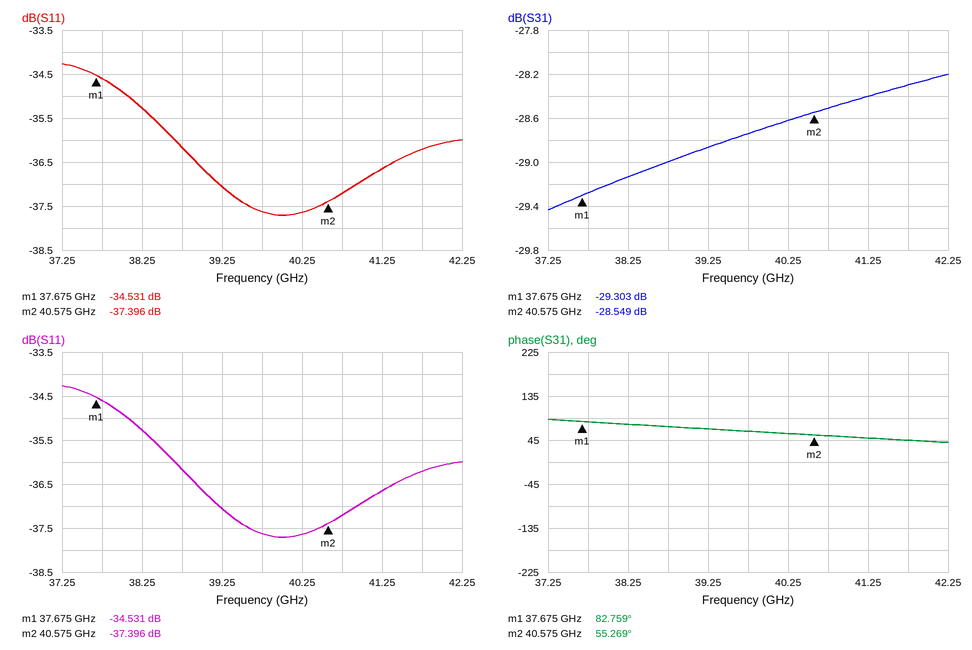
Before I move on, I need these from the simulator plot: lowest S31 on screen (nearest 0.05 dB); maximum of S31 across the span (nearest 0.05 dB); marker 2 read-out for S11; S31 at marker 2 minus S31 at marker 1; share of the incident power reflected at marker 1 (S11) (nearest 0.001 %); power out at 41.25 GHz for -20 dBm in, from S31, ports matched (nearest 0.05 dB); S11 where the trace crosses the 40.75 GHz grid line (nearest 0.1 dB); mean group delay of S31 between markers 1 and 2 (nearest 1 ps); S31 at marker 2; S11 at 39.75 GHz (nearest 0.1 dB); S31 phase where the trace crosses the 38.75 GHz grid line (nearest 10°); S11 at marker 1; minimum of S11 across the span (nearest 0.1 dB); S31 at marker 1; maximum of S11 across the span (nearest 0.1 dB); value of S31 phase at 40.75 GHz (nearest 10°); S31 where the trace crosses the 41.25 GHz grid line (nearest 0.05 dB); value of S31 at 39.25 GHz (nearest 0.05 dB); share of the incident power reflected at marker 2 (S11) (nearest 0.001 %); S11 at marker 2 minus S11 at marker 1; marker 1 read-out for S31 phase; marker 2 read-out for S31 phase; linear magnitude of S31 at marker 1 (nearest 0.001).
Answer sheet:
-29.45 dB
-28.20 dB
-37.396 dB
0.754 dB
0.035 %
-48.40 dBm
-37.2 dB
26 ps
-28.549 dB
-37.6 dB
70°
-34.531 dB
-37.7 dB
-29.303 dB
-34.3 dB
50°
-28.40 dB
-28.85 dB
0.018 %
-2.865 dB
82.759°
55.269°
0.034
